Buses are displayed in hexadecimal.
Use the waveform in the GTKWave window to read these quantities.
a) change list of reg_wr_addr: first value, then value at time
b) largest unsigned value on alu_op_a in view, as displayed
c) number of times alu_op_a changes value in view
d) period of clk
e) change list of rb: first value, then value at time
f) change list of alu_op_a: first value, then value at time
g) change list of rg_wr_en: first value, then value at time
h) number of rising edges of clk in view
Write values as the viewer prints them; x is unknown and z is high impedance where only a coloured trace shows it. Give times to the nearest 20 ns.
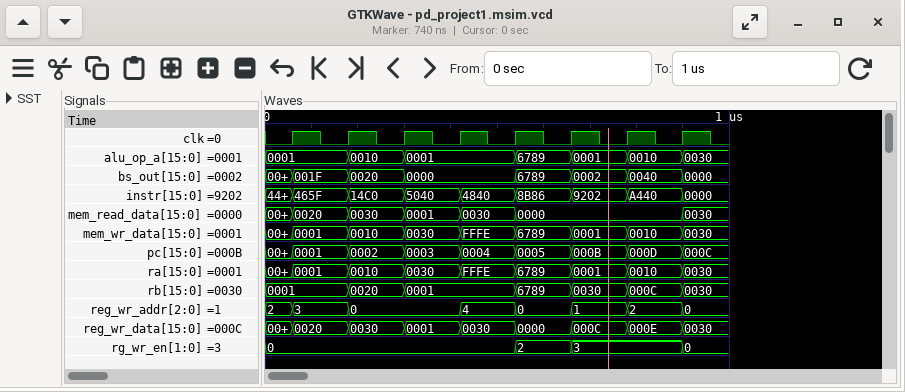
2, 3 at 60 ns, 0 at 180 ns, 4 at 420 ns, 0 at 540 ns, 1 at 660 ns, 2 at 780 ns, 0 at 900 ns
6789
6
120 ns
0001, 0020 at 180 ns, 0001 at 300 ns, 6789 at 540 ns, 0030 at 660 ns, 000C at 780 ns, 0030 at 900 ns
0001, 0010 at 180 ns, 0001 at 300 ns, 6789 at 540 ns, 0001 at 660 ns, 0010 at 780 ns, 0030 at 900 ns
0, 2 at 540 ns, 3 at 660 ns, 0 at 900 ns
8
